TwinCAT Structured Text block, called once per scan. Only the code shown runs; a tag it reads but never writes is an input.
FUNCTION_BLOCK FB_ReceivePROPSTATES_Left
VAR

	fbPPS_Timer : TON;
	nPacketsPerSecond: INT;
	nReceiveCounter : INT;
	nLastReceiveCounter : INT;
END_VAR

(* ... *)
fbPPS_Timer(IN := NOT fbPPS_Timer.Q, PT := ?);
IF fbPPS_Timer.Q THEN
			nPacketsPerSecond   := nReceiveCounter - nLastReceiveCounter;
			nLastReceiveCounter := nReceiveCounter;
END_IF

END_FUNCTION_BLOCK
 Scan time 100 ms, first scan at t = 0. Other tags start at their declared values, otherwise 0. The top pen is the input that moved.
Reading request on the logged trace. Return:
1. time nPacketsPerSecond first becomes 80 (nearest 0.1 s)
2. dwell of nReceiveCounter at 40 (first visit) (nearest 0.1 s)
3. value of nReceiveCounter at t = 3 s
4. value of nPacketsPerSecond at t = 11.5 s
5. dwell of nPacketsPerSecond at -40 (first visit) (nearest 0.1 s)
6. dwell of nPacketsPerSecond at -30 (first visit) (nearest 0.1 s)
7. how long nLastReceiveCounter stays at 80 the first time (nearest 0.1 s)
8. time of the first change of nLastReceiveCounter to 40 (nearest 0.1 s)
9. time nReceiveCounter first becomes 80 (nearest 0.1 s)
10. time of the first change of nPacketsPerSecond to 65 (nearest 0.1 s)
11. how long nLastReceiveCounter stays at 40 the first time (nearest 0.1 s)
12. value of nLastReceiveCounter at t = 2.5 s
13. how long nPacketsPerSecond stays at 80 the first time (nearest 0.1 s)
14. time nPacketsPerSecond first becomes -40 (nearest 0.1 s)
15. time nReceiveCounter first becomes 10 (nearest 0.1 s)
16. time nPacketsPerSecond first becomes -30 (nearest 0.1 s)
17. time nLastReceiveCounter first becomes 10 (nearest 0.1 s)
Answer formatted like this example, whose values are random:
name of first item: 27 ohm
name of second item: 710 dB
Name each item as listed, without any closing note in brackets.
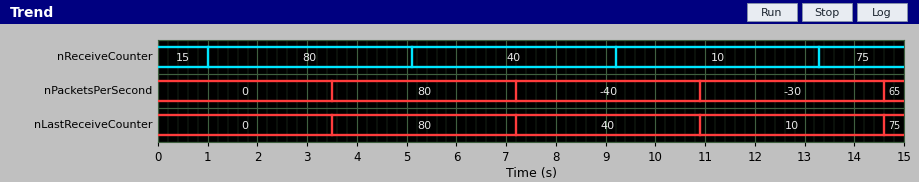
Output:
time nPacketsPerSecond first becomes 80: 3.5 s
dwell of nReceiveCounter at 40 (first visit): 4.1 s
value of nReceiveCounter at t = 3 s: 80
value of nPacketsPerSecond at t = 11.5 s: -30
dwell of nPacketsPerSecond at -40 (first visit): 3.7 s
dwell of nPacketsPerSecond at -30 (first visit): 3.7 s
how long nLastReceiveCounter stays at 80 the first time: 3.7 s
time of the first change of nLastReceiveCounter to 40: 7.2 s
time nReceiveCounter first becomes 80: 1.0 s
time of the first change of nPacketsPerSecond to 65: 14.6 s
how long nLastReceiveCounter stays at 40 the first time: 3.7 s
value of nLastReceiveCounter at t = 2.5 s: 0
how long nPacketsPerSecond stays at 80 the first time: 3.7 s
time nPacketsPerSecond first becomes -40: 7.2 s
time nReceiveCounter first becomes 10: 9.2 s
time nPacketsPerSecond first becomes -30: 10.9 s
time nLastReceiveCounter first becomes 10: 10.9 s
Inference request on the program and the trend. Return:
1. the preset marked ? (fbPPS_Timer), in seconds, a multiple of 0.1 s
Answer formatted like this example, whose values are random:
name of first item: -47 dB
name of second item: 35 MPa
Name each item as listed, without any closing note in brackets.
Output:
the preset marked ? (fbPPS_Timer), in seconds, a multiple of 0.1 s: 3.5 s
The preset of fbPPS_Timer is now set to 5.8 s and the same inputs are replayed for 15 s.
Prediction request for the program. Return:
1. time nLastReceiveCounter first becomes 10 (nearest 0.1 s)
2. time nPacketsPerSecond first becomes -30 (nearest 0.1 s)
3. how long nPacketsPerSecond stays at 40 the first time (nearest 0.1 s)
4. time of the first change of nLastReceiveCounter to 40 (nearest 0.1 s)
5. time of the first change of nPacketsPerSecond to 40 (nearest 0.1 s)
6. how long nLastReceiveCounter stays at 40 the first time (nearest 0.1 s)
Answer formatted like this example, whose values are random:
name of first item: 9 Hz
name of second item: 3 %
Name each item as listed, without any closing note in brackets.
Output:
time nLastReceiveCounter first becomes 10: 11.8 s
time nPacketsPerSecond first becomes -30: 11.8 s
how long nPacketsPerSecond stays at 40 the first time: 6.0 s
time of the first change of nLastReceiveCounter to 40: 5.8 s
time of the first change of nPacketsPerSecond to 40: 5.8 s
how long nLastReceiveCounter stays at 40 the first time: 6.0 s
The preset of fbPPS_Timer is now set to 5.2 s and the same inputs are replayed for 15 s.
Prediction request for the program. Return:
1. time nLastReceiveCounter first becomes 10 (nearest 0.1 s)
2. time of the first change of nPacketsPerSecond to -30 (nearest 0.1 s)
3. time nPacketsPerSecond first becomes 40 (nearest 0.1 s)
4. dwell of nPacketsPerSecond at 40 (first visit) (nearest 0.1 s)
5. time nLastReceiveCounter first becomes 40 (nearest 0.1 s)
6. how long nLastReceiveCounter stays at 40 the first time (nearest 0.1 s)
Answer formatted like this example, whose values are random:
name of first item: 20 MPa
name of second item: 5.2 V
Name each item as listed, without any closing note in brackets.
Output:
time nLastReceiveCounter first becomes 10: 10.6 s
time of the first change of nPacketsPerSecond to -30: 10.6 s
time nPacketsPerSecond first becomes 40: 5.2 s
dwell of nPacketsPerSecond at 40 (first visit): 5.4 s
time nLastReceiveCounter first becomes 40: 5.2 s
how long nLastReceiveCounter stays at 40 the first time: 5.4 s
